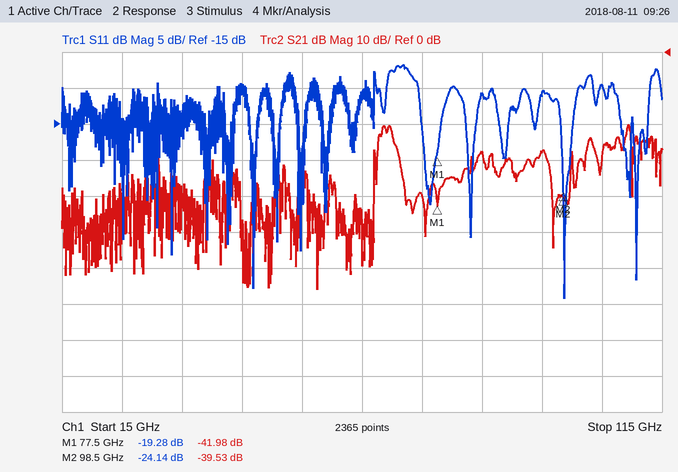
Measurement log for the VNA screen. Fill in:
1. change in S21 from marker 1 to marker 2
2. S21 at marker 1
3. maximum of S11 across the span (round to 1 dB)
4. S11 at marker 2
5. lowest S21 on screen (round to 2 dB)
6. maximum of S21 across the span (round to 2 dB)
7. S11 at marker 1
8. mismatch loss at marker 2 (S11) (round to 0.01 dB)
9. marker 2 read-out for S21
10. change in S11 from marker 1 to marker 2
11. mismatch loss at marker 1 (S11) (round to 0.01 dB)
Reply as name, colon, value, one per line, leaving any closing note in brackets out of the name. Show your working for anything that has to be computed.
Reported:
change in S21 from marker 1 to marker 2: -39.53 − (-41.98) = 2.45 dB
S21 at marker 1: -41.98 dB
maximum of S11 across the span: -7 dB
S11 at marker 2: -24.14 dB
lowest S21 on screen: -66 dB
maximum of S21 across the span: -20 dB
S11 at marker 1: -19.28 dB
mismatch loss at marker 2 (S11): −10 log10(1 − 10^(-24.14/10)) ≈ 0.02 dB
marker 2 read-out for S21: -39.53 dB
change in S11 from marker 1 to marker 2: -24.14 − (-19.28) = -4.86 dB
mismatch loss at marker 1 (S11): −10 log10(1 − 10^(-19.28/10)) ≈ 0.05 dB
